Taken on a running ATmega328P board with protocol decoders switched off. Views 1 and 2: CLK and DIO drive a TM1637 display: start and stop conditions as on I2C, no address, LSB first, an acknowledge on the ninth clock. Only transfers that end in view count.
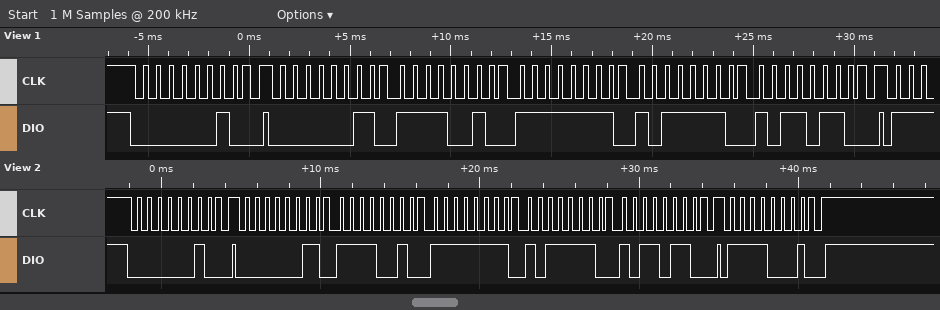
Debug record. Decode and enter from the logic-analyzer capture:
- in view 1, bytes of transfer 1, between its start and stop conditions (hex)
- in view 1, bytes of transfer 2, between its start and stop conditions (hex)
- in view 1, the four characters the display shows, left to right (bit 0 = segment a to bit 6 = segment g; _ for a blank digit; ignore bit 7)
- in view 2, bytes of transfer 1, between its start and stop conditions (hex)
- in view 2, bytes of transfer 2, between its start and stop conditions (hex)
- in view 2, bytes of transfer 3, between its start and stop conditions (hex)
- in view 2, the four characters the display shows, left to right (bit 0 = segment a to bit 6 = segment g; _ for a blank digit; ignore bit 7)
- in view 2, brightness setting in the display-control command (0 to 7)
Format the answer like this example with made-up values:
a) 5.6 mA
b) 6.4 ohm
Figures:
a) 40
b) C0 4F FF 7D 6D
c) 3865
d) 40
e) C0 4F FF 7D 6D
f) 8F
g) 3865
h) 7
